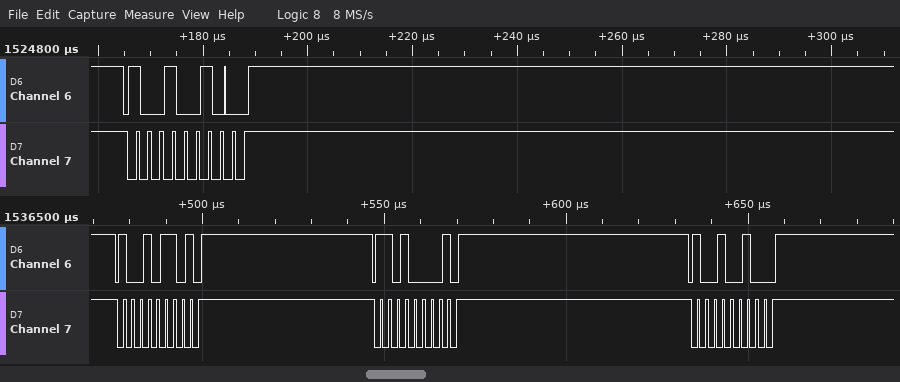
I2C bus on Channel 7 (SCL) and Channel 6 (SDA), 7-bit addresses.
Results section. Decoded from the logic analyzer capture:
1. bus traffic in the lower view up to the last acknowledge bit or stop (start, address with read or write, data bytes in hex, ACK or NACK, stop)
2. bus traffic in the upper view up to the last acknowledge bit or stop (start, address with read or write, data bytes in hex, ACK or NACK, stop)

start, address 4B write NACK, stop, start, address 68 write NACK, stop, start, address 49 write ACK, stop
start, address 49 write ACK, stop
